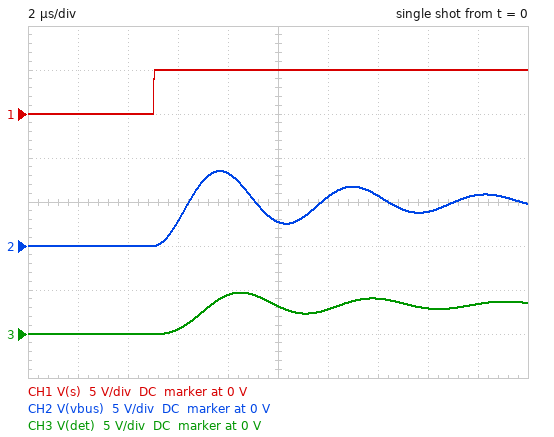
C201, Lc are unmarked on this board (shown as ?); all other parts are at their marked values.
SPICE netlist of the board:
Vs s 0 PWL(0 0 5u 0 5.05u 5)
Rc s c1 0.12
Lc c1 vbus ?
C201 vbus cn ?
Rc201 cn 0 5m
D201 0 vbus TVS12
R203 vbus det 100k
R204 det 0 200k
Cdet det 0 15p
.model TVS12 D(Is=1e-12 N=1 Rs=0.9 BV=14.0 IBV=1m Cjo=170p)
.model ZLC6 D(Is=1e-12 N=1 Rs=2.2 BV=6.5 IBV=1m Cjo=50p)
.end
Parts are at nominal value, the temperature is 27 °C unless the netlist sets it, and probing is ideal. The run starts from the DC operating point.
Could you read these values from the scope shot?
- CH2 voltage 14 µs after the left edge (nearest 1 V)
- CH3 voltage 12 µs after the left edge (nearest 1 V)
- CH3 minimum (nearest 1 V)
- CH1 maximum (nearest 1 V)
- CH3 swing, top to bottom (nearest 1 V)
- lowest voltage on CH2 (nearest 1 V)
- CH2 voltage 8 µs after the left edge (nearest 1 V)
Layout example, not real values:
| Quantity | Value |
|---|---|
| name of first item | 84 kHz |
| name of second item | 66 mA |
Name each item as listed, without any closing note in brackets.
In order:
| Quantity | Value |
|---|---|
| CH2 voltage 14 µs after the left edge | 6 V |
| CH3 voltage 12 µs after the left edge | 3 V |
| CH3 minimum | 0 V |
| CH1 maximum | 5 V |
| CH3 swing, top to bottom | 5 V |
| lowest voltage on CH2 | 0 V |
| CH2 voltage 8 µs after the left edge | 8 V |
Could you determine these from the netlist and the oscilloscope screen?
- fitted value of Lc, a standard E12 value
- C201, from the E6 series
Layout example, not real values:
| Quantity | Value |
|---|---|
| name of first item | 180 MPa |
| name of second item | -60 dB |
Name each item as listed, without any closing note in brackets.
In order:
| Quantity | Value |
|---|---|
| fitted value of Lc, a standard E12 value | 470 nH |
| C201, from the E6 series | 1.5 µF |
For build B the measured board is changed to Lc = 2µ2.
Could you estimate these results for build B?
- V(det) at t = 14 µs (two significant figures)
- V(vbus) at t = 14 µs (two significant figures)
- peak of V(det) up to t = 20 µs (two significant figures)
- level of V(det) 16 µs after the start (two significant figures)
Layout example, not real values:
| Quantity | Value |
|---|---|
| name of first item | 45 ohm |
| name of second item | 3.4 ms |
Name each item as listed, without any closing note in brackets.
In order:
| Quantity | Value |
|---|---|
| V(det) at t = 14 µs | 4.1 V |
| V(vbus) at t = 14 µs | 4.3 V |
| peak of V(det) up to t = 20 µs | 5.8 V |
| level of V(det) 16 µs after the start | 1.8 V |
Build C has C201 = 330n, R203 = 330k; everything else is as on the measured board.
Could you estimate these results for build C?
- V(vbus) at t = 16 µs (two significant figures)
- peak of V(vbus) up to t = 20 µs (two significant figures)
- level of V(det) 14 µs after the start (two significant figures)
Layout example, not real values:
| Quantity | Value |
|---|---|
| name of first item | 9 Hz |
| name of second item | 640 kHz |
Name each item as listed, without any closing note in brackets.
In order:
| Quantity | Value |
|---|---|
| V(vbus) at t = 16 µs | 6.0 V |
| peak of V(vbus) up to t = 20 µs | 9.2 V |
| level of V(det) 14 µs after the start | 2.0 V |
